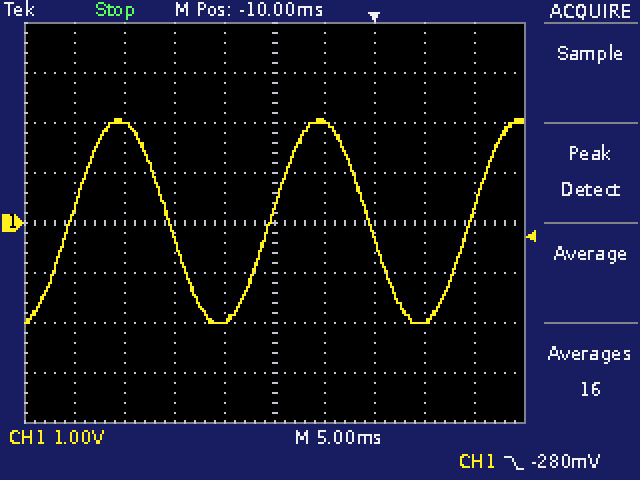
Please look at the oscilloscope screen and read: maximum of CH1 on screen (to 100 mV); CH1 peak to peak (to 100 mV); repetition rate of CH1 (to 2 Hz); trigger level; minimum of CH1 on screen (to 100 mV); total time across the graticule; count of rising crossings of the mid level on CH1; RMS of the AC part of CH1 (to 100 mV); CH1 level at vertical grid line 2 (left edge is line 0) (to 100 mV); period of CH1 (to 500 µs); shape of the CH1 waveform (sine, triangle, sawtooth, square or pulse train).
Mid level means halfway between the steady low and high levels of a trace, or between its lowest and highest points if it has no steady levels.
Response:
2.1 V
4.1 V
50 Hz
-280 mV
-2.0 V
50 ms
3
1.4 V
2.0 V
20.0 ms
sine
